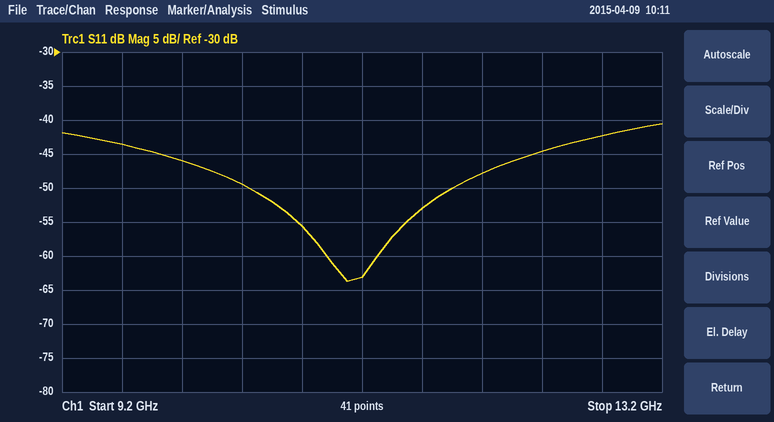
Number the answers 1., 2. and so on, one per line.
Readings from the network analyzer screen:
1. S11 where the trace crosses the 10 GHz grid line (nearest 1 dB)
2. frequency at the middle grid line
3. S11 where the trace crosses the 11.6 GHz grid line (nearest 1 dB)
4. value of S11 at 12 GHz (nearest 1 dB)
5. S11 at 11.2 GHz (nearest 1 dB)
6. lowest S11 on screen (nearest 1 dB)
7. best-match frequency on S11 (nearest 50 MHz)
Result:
1. -46 dB
2. 11.2 GHz
3. -53 dB
4. -48 dB
5. -63 dB
6. -64 dB
7. 11.10 GHz
